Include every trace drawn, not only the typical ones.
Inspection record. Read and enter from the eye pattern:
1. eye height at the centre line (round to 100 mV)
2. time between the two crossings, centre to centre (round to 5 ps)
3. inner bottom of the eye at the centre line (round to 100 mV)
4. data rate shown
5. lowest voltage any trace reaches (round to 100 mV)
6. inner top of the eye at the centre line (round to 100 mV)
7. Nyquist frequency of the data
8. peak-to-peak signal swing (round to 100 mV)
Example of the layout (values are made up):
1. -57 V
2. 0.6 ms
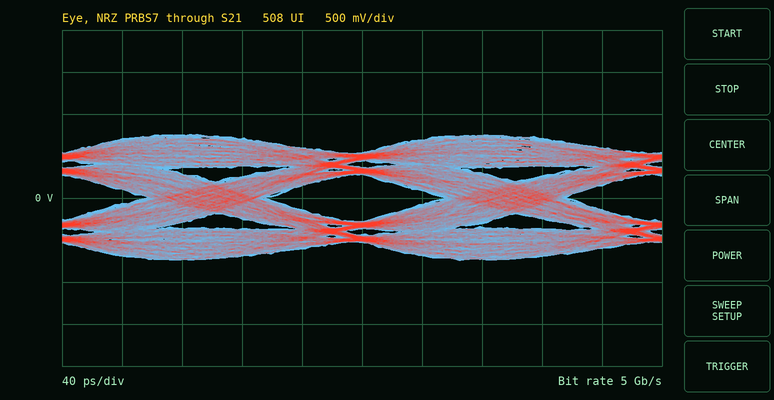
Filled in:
1. 600 mV
2. 200 ps
3. -300 mV
4. 5 Gb/s
5. -700 mV
6. 300 mV
7. 2.5 GHz
8. 1.5 V
